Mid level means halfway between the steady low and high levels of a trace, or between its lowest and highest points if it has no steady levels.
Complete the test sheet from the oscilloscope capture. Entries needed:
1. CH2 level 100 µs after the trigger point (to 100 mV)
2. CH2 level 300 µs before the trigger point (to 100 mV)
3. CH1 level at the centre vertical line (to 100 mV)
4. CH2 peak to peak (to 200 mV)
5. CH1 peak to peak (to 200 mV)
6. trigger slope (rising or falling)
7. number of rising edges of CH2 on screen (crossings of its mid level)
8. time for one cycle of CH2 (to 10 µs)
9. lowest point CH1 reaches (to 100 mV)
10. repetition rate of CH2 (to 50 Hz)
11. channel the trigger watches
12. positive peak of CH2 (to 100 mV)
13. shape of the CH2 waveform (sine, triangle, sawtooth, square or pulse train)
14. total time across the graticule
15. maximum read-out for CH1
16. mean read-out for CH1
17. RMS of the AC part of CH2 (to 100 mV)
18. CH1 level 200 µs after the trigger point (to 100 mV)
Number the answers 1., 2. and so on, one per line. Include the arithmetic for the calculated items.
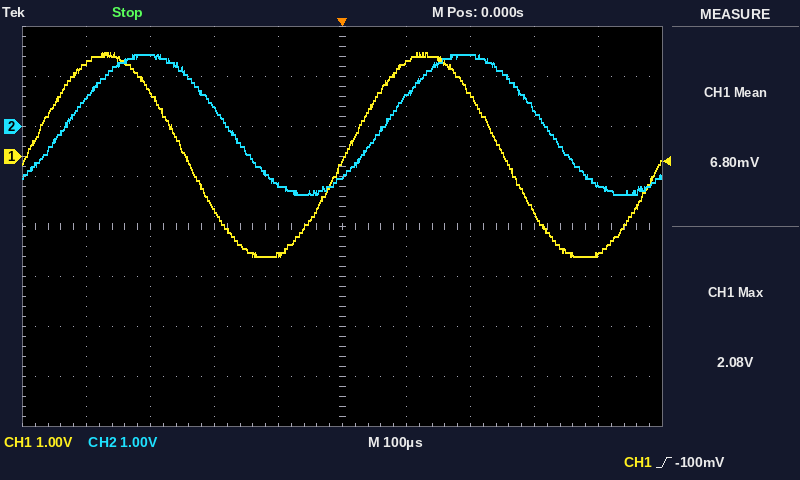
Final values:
1. 600 mV
2. 1.4 V
3. -100 mV
4. 2.8 V
5. 4.0 V
6. rising
7. 2
8. 500 µs
9. -2.0 V
10. 1 / 500 µs ≈ 2.00 kHz
11. CH1
12. 1.4 V
13. sine
14. 1 ms
15. 2.08 V
16. 6.80 mV
17. 2.8 V / (2√2) ≈ 1.0 V
18. 1.2 V
